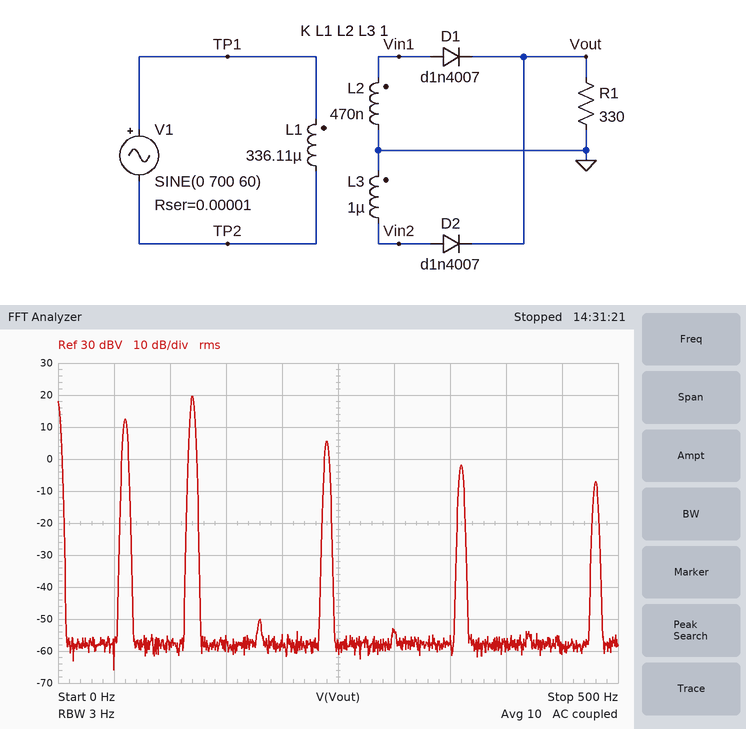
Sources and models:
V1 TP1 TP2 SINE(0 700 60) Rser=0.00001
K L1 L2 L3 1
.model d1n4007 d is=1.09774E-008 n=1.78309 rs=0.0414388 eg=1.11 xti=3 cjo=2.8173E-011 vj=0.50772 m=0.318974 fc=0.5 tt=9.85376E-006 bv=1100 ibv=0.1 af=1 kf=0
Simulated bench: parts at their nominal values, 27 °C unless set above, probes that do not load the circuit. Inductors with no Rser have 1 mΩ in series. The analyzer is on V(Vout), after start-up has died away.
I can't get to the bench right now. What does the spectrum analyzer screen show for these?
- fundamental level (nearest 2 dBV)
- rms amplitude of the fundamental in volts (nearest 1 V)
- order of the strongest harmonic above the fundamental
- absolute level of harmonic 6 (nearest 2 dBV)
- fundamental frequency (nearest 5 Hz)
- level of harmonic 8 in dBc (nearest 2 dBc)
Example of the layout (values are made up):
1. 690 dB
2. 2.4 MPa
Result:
1. 12 dBV
2. 4 V
3. 2
4. -2 dBV
5. 60 Hz
6. -20 dBc
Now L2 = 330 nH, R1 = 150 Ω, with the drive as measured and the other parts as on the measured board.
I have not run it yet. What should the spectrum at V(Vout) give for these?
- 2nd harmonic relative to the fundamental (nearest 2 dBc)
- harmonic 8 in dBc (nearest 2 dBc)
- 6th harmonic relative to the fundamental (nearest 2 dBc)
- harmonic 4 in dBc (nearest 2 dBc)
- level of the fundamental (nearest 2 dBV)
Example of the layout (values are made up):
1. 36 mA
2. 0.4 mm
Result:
1. 4 dBc
2. -22 dBc
3. -18 dBc
4. -10 dBc
5. 16 dBV
